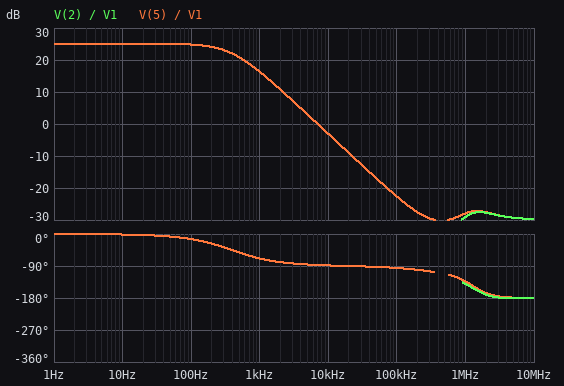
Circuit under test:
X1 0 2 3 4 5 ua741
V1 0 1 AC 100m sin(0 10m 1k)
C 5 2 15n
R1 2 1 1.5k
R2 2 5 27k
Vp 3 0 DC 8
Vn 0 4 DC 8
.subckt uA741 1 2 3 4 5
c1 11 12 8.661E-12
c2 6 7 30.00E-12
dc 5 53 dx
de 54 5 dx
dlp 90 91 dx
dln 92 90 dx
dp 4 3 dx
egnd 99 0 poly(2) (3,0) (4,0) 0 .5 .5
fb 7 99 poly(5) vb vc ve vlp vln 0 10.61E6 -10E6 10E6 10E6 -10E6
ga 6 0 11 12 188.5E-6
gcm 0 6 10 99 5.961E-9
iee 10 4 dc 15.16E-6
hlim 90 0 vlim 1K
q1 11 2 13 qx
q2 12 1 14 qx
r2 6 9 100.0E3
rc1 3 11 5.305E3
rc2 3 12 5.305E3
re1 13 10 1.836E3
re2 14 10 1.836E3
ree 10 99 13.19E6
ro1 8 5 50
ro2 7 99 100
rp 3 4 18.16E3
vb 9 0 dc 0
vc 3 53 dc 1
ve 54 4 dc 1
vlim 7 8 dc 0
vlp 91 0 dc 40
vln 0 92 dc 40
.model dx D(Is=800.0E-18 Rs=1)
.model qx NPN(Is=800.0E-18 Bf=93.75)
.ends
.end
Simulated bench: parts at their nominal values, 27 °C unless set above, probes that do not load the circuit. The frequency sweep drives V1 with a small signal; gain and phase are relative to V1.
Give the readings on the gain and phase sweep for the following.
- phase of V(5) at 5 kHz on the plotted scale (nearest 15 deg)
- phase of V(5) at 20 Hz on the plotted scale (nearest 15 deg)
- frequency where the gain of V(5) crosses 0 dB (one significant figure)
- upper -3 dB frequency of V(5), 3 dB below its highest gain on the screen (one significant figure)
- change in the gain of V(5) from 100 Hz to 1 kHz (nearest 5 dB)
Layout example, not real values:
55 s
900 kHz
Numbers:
-90 deg
0 deg
7 kHz
400 Hz
-10 dB
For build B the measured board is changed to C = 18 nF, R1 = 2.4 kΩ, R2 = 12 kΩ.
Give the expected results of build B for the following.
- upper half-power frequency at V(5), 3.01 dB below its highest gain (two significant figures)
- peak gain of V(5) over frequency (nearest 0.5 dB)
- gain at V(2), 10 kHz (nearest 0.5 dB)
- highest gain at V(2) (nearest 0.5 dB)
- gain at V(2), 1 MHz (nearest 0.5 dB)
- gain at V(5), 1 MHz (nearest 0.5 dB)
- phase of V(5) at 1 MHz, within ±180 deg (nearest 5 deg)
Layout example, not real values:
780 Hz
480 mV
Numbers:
730 Hz
14.0 dB
-48.5 dB
-31.5 dB
-33.0 dB
-32.0 dB
-130 deg
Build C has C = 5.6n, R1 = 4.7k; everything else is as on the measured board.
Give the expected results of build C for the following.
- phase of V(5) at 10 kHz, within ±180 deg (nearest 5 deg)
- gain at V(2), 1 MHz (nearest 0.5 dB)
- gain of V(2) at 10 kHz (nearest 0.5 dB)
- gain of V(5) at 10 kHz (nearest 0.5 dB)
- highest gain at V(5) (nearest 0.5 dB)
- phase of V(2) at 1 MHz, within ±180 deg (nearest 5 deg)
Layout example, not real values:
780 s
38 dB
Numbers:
-85 deg
-38.0 dB
-44.5 dB
-4.5 dB
15.0 dB
-155 deg
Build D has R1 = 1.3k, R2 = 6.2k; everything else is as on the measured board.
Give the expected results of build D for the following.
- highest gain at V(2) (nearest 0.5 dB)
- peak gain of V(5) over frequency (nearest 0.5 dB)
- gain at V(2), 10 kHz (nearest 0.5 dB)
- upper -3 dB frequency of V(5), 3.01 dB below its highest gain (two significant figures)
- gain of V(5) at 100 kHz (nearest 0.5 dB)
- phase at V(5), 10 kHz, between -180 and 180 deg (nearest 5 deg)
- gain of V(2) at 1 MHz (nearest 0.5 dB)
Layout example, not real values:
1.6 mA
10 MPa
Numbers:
-26.5 dB
13.5 dB
-42.0 dB
1.7 kHz
-21.5 dB
-80 deg
-28.0 dB
